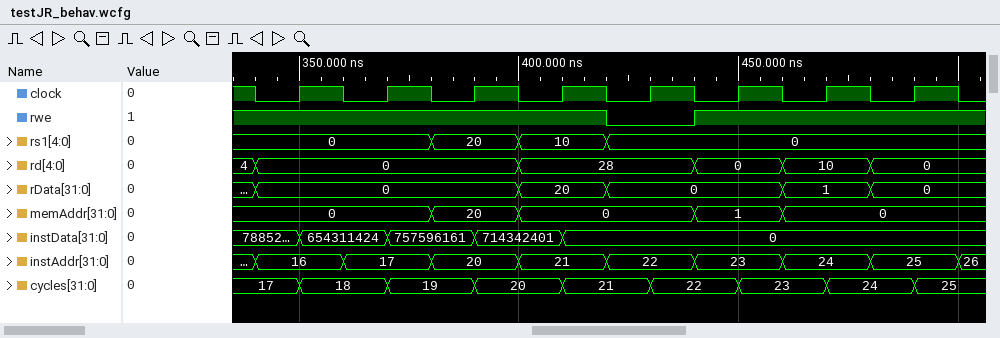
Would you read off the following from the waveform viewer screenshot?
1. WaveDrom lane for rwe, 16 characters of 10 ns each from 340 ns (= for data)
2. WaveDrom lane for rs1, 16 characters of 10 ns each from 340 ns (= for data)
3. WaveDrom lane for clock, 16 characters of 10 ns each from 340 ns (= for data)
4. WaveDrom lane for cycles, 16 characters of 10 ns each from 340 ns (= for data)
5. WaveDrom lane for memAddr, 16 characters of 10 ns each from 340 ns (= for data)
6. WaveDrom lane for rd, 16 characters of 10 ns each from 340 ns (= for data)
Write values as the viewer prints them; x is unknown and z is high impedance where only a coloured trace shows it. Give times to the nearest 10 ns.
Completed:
{name: 'rwe', wave: '1.......0.1.....'}
{name: 'rs1', wave: '=...=.=.=.......', data: '0 20 10 0'}
{name: 'clock', wave: '0101010101010101'}
{name: 'cycles', wave: '==.=.=.=.=.=.=.=', data: '17 18 19 20 21 22 23 24 25'}
{name: 'memAddr', wave: '=...=.=...=.=...', data: '0 20 0 1 0'}
{name: 'rd', wave: '=.....=...=.=.=.', data: '0 28 0 10 0'}
